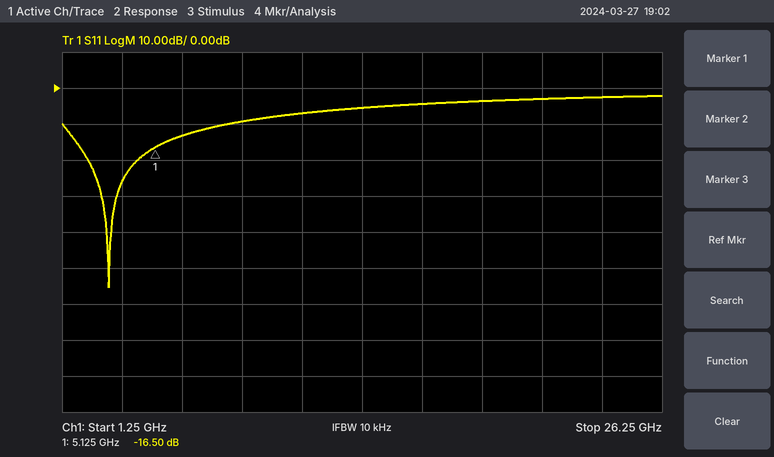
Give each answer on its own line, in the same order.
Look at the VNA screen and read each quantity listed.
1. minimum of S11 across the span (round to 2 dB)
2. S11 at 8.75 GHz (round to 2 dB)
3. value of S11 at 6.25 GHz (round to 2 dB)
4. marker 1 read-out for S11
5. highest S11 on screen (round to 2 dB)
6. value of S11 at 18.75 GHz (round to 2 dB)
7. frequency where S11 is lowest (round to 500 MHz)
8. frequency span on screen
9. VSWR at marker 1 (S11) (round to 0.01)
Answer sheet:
-56 dB
-10 dB
-14 dB
-16.50 dB
-2 dB
-4 dB
3.0 GHz
25 GHz
1.35
